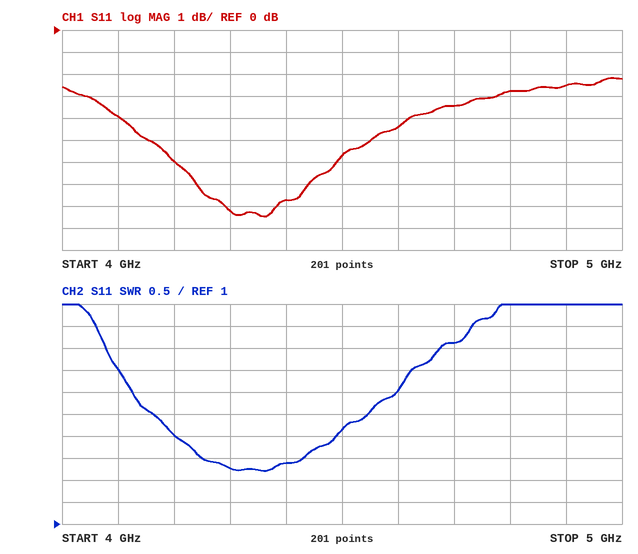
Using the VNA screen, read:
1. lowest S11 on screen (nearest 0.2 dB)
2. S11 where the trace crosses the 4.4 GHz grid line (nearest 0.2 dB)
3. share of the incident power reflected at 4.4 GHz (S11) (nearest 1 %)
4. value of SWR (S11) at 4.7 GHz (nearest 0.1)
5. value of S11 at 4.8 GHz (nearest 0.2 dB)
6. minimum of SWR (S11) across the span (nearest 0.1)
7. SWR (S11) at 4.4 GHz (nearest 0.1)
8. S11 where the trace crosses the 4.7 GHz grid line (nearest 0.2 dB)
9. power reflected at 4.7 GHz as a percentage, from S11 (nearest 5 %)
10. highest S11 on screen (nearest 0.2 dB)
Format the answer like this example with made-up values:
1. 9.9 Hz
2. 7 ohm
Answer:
1. -8.4 dB
2. -7.8 dB
3. 17 %
4. 5.1
5. -2.8 dB
6. 2.2
7. 2.4
8. -3.4 dB
9. 45 %
10. -2.2 dB
